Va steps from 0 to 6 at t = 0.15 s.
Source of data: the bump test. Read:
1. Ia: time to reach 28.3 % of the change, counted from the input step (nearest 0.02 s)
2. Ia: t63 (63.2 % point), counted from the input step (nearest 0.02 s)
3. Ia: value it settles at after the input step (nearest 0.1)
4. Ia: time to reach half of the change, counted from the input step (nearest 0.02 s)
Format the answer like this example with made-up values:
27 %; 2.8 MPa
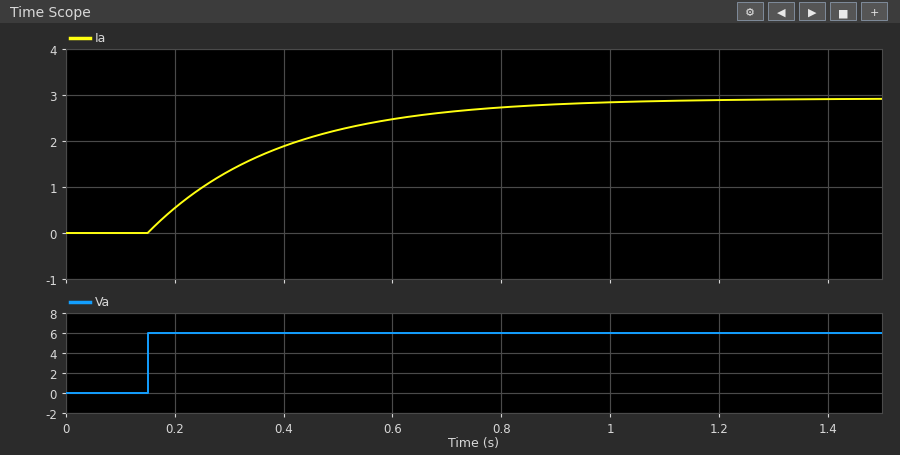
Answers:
0.08 s; 0.24 s; 2.9; 0.16 s
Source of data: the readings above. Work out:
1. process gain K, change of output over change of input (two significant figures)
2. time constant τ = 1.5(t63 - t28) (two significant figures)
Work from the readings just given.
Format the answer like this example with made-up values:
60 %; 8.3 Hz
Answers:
0.48; 0.24 s
